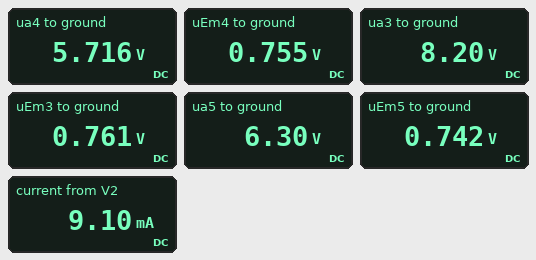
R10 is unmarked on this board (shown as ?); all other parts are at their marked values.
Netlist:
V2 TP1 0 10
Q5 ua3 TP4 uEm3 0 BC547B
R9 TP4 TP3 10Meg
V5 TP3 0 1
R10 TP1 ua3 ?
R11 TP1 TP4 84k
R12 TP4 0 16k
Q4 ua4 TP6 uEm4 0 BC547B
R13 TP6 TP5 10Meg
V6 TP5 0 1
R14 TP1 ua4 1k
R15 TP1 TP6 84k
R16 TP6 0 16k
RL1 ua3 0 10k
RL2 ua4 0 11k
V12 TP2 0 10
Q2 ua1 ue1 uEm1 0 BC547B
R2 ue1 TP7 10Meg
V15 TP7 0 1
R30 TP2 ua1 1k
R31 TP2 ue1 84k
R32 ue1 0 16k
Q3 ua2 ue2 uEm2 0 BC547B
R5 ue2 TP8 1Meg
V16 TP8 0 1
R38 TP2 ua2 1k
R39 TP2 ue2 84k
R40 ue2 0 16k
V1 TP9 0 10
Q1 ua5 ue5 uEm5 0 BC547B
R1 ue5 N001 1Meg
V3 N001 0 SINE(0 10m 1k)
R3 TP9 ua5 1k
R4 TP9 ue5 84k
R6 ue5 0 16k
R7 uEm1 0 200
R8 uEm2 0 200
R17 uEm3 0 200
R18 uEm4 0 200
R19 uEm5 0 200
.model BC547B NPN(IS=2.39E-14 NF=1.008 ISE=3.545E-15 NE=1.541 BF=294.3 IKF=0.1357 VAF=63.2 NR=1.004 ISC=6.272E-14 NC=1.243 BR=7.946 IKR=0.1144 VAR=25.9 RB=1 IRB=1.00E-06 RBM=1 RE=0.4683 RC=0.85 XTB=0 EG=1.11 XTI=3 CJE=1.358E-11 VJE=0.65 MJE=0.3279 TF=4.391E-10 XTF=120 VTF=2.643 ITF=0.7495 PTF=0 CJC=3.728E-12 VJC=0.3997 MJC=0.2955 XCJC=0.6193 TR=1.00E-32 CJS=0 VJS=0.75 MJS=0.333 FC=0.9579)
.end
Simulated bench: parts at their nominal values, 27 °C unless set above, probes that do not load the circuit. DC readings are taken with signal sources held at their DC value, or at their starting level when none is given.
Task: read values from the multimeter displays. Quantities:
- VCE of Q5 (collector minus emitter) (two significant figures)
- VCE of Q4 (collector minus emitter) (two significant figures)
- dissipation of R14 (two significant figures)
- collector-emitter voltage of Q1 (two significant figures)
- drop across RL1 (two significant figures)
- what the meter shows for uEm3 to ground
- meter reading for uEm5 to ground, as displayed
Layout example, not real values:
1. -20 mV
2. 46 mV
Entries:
1. 7.4 V
2. 5.0 V
3. 18 mW
4. 5.6 V
5. 8.2 V
6. 0.761 V
7. 0.742 V
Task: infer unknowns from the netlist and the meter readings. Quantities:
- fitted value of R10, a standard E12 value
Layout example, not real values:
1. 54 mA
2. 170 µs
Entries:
1. 390 Ω
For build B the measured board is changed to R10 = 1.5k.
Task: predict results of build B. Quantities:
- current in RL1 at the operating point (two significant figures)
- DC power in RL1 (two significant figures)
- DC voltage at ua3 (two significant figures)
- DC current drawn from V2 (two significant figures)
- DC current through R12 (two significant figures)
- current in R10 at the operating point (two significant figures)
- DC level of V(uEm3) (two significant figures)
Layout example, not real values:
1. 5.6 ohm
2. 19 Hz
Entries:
1. 380 µA
2. 1.5 mW
3. 3.8 V
4. 8.6 mA
5. 89 µA
6. 4.1 mA
7. 750 mV
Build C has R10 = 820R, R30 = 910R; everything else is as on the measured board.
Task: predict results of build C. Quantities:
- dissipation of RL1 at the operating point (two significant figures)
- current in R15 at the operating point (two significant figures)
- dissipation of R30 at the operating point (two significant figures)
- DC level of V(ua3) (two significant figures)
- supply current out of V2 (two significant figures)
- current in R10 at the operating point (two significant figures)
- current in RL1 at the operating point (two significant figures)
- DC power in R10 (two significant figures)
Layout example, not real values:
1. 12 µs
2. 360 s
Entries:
1. 4.1 mW
2. 100 µA
3. 13 mW
4. 6.4 V
5. 8.9 mA
6. 4.4 mA
7. 640 µA
8. 16 mW
